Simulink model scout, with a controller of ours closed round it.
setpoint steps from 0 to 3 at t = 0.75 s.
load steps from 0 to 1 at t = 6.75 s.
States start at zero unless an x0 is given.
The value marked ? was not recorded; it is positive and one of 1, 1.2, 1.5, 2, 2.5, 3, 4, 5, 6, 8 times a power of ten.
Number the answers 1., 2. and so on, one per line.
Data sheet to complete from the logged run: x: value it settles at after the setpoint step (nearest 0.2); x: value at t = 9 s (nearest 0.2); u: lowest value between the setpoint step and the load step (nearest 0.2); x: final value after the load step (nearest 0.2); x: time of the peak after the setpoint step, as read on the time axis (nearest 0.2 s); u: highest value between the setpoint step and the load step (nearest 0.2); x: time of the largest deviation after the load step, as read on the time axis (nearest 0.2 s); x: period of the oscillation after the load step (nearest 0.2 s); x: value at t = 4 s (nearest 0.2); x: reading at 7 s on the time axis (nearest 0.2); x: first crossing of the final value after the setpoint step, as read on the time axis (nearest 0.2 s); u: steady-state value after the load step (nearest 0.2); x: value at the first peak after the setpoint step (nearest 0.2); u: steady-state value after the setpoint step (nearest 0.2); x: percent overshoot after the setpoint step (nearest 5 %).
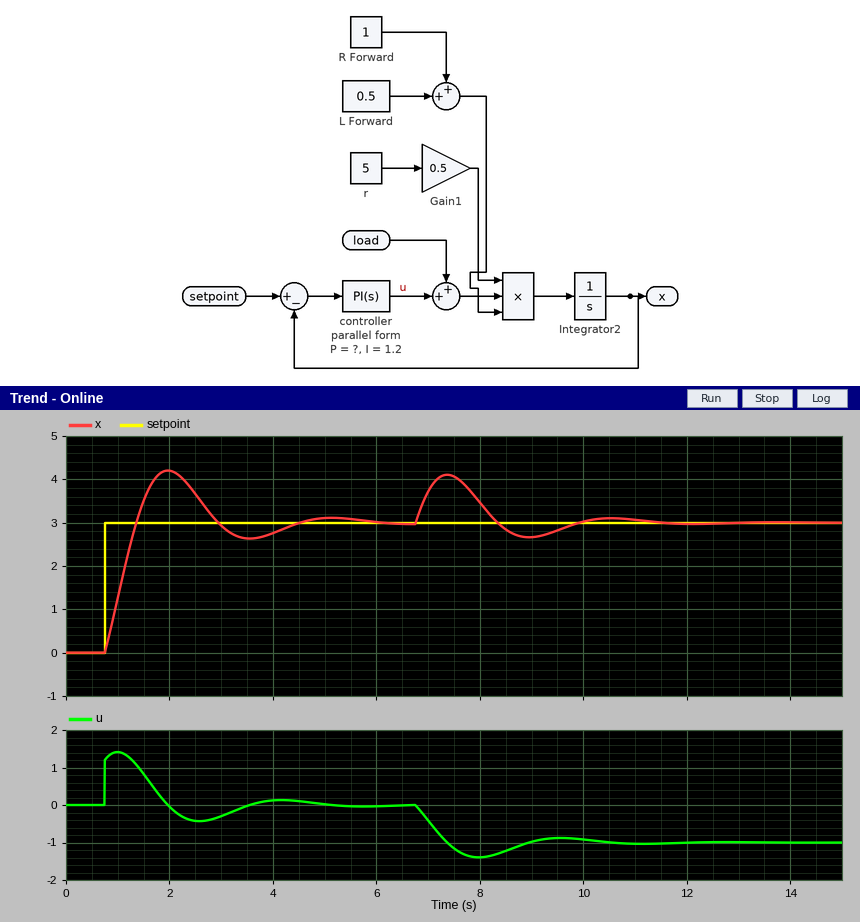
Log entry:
1. 3.0
2. 2.6
3. -0.4
4. 3.0
5. 2.0 s
6. 1.4
7. 7.4 s
8. 3.2 s
9. 2.8
10. 3.8
11. 1.4 s
12. -1.0
13. 4.2
14. 0.0
15. 40 %
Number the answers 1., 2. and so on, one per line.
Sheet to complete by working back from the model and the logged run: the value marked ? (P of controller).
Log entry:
1. 0.4
